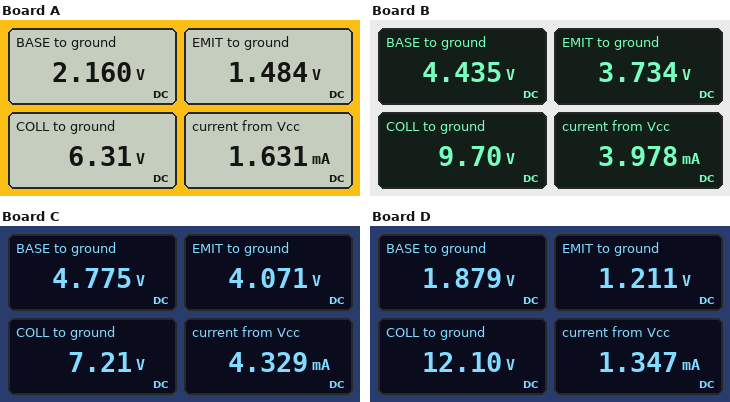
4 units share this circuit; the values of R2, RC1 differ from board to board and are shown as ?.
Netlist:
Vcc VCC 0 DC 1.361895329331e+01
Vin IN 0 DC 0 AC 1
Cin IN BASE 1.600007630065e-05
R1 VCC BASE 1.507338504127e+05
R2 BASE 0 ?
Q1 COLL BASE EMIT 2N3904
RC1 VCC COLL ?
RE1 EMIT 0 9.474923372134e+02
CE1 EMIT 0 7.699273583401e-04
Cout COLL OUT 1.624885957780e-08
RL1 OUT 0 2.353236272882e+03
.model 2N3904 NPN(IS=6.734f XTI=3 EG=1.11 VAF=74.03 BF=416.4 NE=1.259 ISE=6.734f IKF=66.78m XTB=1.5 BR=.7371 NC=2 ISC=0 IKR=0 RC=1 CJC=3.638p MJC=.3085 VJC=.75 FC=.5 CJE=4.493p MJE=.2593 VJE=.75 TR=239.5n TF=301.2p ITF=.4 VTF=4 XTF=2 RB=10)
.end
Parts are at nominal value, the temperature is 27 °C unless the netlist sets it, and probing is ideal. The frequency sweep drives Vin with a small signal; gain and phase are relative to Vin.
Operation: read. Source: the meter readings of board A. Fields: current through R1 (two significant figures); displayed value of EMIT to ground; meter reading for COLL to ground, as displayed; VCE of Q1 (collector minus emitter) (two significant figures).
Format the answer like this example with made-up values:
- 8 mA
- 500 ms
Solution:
- 76 µA
- 1.484 V
- 6.31 V
- 4.8 V
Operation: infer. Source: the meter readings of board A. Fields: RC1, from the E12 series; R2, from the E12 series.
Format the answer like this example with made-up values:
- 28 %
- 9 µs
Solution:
- 4.7 kΩ
- 33 kΩ
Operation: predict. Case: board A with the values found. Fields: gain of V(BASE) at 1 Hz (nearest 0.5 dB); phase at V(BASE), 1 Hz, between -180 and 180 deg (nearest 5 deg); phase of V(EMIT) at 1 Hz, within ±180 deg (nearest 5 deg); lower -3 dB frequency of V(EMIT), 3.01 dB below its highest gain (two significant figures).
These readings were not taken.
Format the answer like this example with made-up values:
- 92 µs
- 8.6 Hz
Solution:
- -3.0 dB
- 20 deg
- 15 deg
- 320 mHz
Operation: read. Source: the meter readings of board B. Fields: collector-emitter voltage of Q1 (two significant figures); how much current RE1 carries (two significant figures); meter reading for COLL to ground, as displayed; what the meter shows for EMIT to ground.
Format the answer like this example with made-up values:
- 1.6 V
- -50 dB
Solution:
- 6.0 V
- 3.9 mA
- 9.70 V
- 3.734 V
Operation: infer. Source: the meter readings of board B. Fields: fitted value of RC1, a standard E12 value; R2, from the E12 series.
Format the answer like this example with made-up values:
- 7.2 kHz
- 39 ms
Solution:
- 1 kΩ
- 120 kΩ
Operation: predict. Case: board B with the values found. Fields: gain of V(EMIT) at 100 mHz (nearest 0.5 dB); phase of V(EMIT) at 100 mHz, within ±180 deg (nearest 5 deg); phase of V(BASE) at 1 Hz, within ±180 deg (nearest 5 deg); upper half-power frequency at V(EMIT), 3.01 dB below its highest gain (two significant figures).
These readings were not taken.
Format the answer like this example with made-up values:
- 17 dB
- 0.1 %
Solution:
- -8.0 dB
- 60 deg
- 10 deg
- 37 Hz
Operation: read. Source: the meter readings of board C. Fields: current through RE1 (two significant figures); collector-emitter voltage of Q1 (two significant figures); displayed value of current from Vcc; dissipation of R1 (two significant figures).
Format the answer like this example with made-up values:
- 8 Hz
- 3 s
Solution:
- 4.3 mA
- 3.1 V
- 4.329 mA
- 520 µW
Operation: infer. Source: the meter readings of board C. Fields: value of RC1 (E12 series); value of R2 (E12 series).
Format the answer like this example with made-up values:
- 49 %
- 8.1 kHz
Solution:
- 1.5 kΩ
- 150 kΩ
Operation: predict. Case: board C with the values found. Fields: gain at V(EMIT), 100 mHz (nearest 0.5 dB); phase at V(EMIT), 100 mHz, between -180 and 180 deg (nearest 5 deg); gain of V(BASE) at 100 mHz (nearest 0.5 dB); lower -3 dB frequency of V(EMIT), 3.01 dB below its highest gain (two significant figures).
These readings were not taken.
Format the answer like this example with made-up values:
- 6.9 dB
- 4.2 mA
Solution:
- -7.5 dB
- 55 deg
- -7.5 dB
- 150 mHz
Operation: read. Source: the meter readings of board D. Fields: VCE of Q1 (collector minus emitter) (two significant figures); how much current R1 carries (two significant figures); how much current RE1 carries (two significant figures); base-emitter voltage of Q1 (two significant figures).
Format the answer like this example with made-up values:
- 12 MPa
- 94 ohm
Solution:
- 11 V
- 78 µA
- 1.3 mA
- 670 mV
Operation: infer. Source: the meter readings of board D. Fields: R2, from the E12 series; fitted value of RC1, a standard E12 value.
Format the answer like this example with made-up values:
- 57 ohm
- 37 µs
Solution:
- 27 kΩ
- 1.2 kΩ
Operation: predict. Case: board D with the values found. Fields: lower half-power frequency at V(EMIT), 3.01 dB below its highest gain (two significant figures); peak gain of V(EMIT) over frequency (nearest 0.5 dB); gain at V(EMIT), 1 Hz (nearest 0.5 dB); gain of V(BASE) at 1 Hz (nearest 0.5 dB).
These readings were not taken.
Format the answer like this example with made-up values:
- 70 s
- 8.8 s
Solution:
- 370 mHz
- -2.5 dB
- -3.0 dB
- -2.5 dB
